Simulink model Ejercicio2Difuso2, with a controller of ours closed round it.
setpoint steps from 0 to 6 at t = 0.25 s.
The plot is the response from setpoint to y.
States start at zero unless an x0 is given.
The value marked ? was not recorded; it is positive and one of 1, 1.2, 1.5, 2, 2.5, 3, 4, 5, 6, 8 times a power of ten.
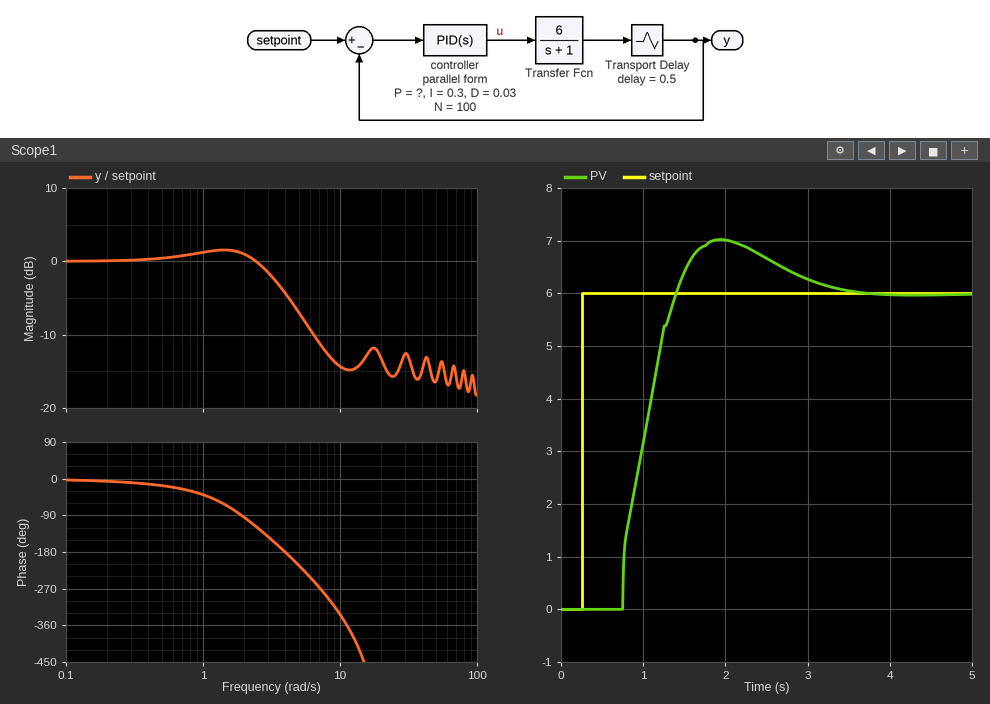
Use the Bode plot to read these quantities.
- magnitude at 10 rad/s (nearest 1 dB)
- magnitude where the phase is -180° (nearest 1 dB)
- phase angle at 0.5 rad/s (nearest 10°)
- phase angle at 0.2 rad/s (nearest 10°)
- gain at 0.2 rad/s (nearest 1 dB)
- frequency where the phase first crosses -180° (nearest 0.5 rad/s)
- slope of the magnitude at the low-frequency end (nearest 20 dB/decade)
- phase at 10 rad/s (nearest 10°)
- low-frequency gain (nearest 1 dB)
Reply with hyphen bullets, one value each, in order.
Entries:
- -14 dB
- -4 dB
- -20°
- -10°
- 0 dB
- 4.0 rad/s
- 0 dB/decade
- -330°
- 0 dB
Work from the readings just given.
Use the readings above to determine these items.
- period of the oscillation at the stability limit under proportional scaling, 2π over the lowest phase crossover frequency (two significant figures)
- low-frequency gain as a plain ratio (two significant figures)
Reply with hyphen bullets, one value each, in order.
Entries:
- 1.6 s
- 1.0
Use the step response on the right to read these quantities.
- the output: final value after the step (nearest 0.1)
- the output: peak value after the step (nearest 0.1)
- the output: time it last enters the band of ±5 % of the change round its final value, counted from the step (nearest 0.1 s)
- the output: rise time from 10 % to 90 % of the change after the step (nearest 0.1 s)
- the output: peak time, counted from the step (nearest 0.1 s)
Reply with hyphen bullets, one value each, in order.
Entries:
- 6.0
- 7.0
- 2.7 s
- 0.5 s
- 1.7 s
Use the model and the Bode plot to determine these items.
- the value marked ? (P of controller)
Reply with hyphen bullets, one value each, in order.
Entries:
- 0.25
